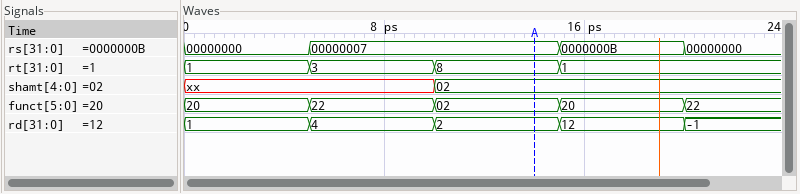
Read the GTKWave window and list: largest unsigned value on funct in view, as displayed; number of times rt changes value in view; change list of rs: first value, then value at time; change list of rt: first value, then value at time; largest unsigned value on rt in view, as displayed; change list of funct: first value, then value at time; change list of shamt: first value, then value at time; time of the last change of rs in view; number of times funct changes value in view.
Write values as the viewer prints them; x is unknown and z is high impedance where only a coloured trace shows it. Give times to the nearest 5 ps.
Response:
22
3
00000000, 00000007 at 5 ps, 0000000B at 15 ps, 00000000 at 20 ps
1, 3 at 5 ps, 8 at 10 ps, 1 at 15 ps
8
20, 22 at 5 ps, 02 at 10 ps, 20 at 15 ps, 22 at 20 ps
xx, 02 at 10 ps
20 ps
4
